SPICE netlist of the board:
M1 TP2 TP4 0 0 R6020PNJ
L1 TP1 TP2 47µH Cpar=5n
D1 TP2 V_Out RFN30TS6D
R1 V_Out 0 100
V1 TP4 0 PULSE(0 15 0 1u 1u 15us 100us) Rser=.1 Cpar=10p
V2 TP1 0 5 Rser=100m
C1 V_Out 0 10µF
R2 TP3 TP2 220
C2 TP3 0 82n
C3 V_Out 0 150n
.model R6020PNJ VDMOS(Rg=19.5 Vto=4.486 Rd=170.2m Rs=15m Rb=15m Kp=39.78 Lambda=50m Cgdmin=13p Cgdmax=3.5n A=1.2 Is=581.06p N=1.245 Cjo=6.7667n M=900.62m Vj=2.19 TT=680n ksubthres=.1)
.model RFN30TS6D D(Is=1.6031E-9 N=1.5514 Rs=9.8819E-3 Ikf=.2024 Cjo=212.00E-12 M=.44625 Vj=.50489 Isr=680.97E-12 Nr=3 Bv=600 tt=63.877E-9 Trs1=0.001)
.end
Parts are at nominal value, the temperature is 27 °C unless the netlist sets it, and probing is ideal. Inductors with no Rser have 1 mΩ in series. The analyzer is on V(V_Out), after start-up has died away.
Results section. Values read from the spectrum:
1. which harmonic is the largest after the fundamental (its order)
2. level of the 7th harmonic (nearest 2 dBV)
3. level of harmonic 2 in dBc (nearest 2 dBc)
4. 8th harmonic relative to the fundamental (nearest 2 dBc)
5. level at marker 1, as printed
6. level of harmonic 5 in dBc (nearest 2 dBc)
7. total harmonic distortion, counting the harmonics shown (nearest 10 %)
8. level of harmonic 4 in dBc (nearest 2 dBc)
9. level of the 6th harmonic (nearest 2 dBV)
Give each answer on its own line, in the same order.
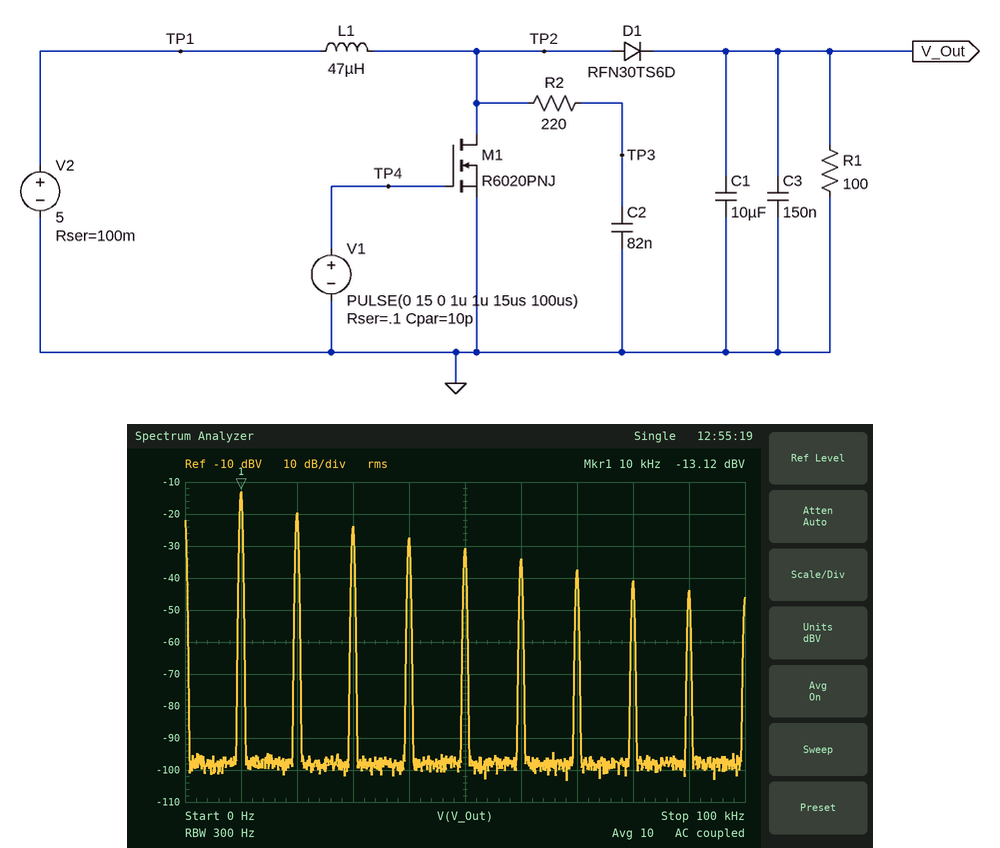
2
-38 dBV
-6 dBc
-28 dBc
-13.12 dBV
-18 dBc
60 %
-14 dBc
-34 dBV
